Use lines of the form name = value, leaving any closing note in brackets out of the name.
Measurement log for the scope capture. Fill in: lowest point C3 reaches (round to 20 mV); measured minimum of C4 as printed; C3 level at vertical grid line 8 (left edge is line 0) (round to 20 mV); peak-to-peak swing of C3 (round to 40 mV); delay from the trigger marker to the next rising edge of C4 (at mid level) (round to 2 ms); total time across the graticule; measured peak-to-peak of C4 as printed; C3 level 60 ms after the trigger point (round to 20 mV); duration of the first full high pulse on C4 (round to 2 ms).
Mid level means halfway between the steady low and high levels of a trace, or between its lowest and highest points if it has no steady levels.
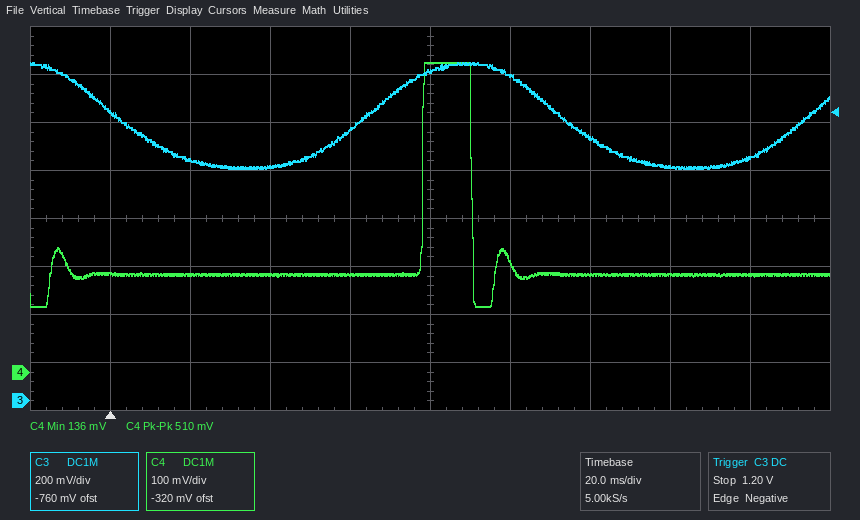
lowest point C3 reaches = 960 mV
measured minimum of C4 as printed = 136 mV
C3 level at vertical grid line 8 (left edge is line 0) = 980 mV
peak-to-peak swing of C3 = 440 mV
delay from the trigger marker to the next rising edge of C4 (at mid level) = 78 ms
total time across the graticule = 200 ms
measured peak-to-peak of C4 as printed = 510 mV
C3 level 60 ms after the trigger point = 1.12 V
duration of the first full high pulse on C4 = 12 ms
